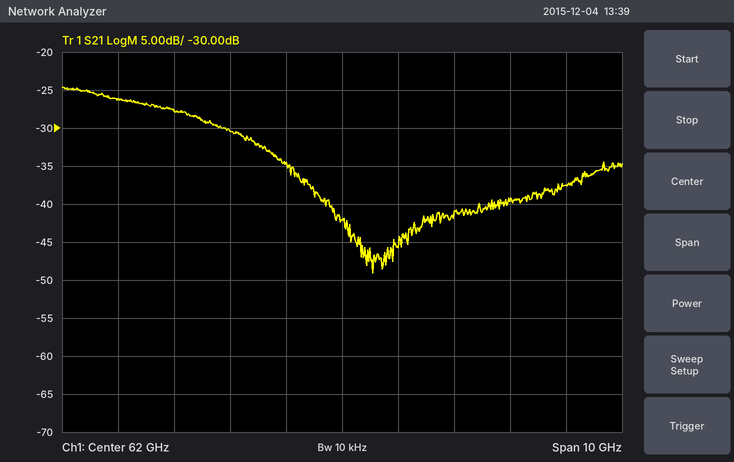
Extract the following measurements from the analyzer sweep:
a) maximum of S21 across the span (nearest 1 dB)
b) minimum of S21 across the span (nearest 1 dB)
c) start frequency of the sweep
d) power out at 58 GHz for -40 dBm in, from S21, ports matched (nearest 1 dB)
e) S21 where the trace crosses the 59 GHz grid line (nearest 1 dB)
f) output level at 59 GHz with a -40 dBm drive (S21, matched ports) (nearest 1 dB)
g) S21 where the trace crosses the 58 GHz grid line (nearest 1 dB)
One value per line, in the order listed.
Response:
-25 dB
-49 dB
57 GHz
-66 dBm
-28 dB
-68 dBm
-26 dB
